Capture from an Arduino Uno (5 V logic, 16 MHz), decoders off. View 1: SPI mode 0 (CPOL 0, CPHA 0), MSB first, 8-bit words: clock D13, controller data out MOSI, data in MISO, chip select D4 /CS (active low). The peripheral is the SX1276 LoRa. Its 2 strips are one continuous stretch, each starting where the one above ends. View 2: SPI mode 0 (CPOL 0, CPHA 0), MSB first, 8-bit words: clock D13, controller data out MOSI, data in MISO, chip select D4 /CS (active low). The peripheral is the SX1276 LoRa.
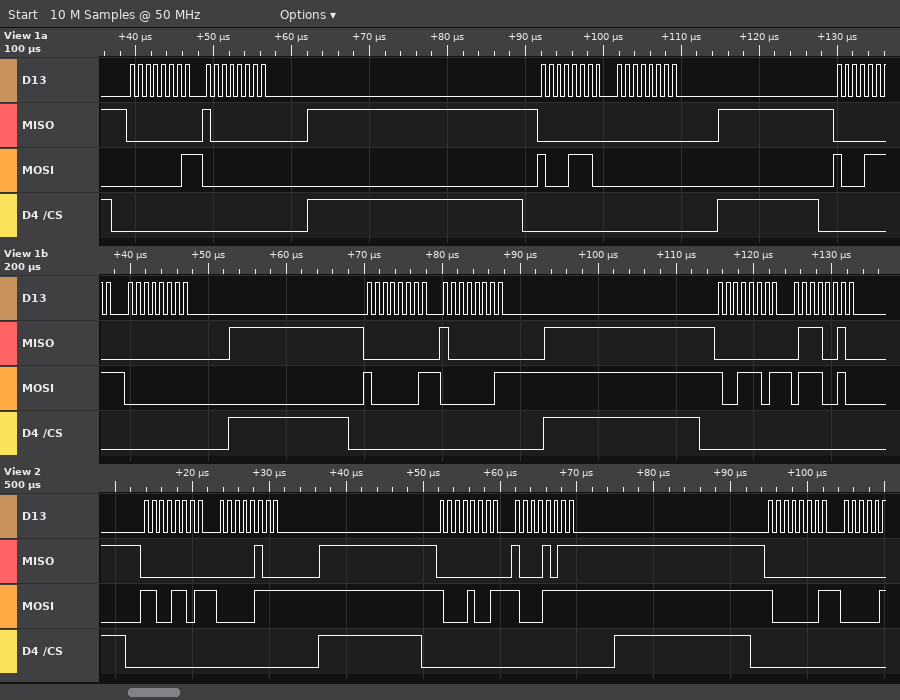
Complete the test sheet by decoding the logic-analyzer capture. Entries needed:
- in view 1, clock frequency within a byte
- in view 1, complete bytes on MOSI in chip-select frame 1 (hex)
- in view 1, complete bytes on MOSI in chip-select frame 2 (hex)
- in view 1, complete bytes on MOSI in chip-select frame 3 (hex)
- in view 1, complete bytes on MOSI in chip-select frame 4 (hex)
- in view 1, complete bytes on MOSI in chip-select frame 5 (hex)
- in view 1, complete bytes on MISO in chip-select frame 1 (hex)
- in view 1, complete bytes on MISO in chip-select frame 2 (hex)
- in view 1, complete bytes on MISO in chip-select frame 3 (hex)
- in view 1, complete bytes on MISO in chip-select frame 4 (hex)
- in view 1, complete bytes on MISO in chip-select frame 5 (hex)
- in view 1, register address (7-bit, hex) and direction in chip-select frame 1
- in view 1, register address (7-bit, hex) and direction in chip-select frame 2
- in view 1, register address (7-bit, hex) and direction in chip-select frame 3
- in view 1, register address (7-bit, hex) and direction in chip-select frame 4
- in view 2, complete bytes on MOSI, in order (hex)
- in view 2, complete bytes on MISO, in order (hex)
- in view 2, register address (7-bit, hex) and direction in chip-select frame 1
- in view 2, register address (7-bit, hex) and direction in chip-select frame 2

1 MHz
01 00
8E 00
8F 00
81 01
9D 72
00 80
00 00
00 00
00 80
00 72
0x01 read
0x0E write
0x0F write
0x01 write
0xCD 0x07 0x89 0x8F 0x81
0x00 0x04 0x00 0x8B 0x00
0x4D write
0x09 write
